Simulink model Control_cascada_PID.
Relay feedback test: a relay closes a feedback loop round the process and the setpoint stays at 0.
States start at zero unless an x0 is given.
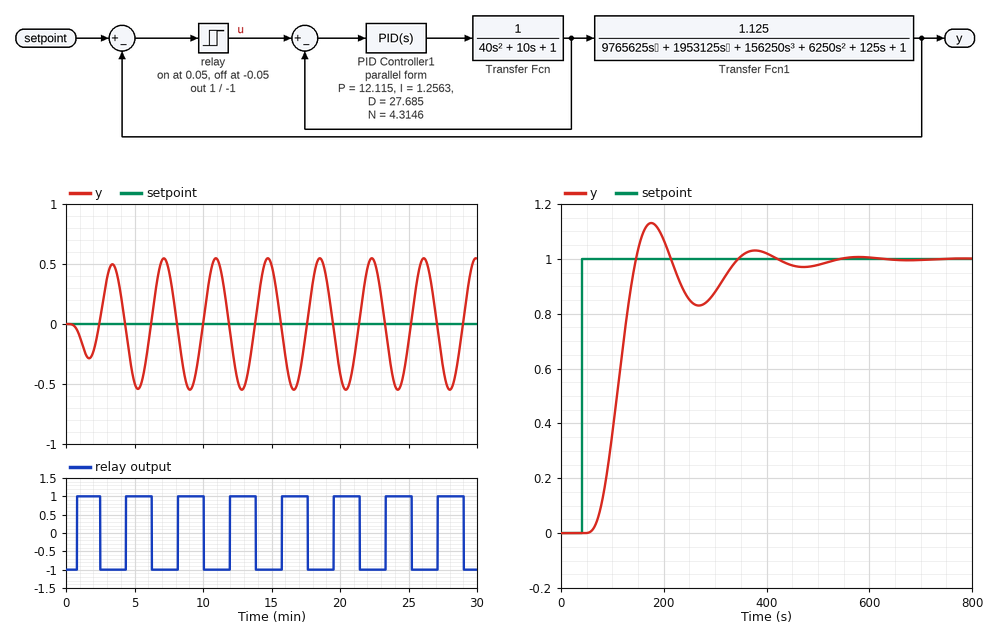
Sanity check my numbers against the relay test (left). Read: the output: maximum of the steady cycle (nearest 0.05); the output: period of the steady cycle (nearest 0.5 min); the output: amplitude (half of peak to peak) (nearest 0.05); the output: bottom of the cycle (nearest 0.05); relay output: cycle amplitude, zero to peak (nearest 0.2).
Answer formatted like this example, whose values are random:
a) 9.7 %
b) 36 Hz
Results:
a) 0.55
b) 4.0 min
c) 0.55
d) -0.55
e) 1.0
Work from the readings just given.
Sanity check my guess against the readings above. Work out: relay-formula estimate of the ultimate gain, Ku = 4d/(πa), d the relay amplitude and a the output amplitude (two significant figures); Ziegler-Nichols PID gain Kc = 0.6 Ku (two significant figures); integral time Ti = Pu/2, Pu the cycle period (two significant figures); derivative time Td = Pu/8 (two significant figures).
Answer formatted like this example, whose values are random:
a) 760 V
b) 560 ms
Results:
a) 2.3
b) 1.4
c) 2.0 min
d) 0.50 min
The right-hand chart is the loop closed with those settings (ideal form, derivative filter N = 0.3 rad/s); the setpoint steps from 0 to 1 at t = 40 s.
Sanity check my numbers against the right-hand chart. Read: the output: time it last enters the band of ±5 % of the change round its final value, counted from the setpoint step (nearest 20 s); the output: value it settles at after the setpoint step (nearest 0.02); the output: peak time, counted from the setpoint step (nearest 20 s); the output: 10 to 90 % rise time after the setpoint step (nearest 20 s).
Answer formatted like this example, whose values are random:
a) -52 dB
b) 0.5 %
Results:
a) 280 s
b) 1.00
c) 140 s
d) 60 s
